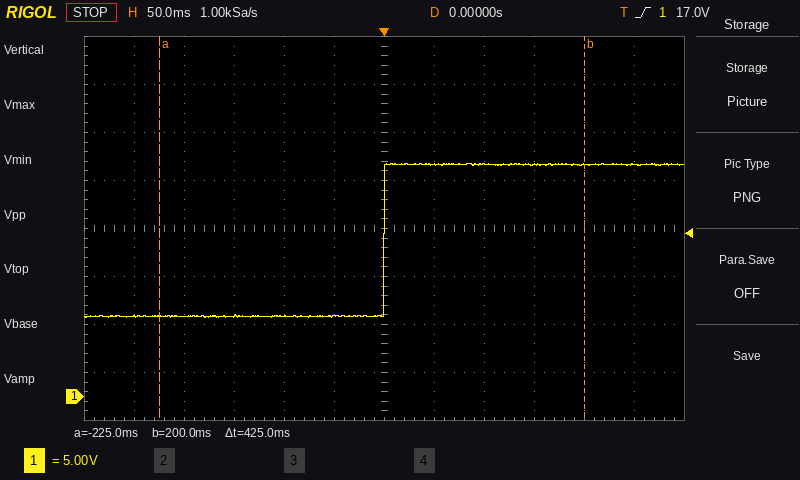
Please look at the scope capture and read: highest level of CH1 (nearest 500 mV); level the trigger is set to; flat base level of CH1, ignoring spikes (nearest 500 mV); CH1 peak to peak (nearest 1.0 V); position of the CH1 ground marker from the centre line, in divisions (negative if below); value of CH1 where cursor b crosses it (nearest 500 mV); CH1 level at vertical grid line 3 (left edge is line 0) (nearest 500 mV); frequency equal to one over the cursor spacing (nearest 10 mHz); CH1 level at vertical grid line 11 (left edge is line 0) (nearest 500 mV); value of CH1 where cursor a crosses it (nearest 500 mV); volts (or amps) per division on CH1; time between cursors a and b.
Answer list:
24.5 V
17.0 V
8.5 V
16.0 V
-3.5 div
24.0 V
8.5 V
2.35 Hz
24.0 V
8.5 V
5 V
425 ms
